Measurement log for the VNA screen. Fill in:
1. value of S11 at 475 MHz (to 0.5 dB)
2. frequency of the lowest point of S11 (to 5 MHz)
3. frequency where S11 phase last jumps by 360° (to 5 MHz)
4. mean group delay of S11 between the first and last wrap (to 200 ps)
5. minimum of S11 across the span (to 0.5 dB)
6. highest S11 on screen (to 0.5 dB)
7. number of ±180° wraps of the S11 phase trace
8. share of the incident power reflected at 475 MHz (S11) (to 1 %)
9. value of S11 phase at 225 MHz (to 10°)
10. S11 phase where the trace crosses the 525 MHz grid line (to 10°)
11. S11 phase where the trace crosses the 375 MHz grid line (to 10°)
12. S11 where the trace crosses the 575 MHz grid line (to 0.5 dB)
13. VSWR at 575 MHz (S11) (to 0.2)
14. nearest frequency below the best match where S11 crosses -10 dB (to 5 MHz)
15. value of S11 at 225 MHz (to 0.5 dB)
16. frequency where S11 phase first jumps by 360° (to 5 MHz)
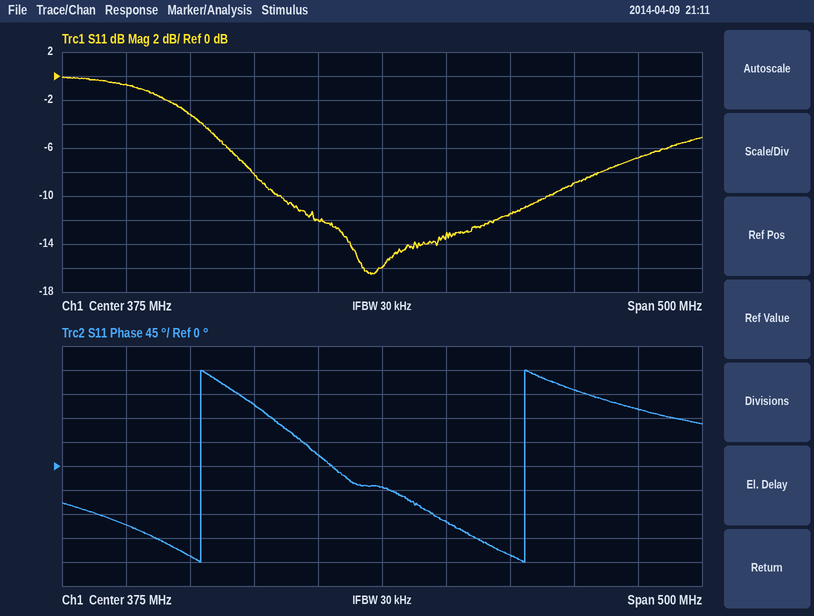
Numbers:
-11.5 dB
365 MHz
485 MHz
4.0 ns
-16.5 dB
0.0 dB
2
7 %
-170°
140°
-40°
-7.0 dB
2.6
295 MHz
-3.0 dB
235 MHz
